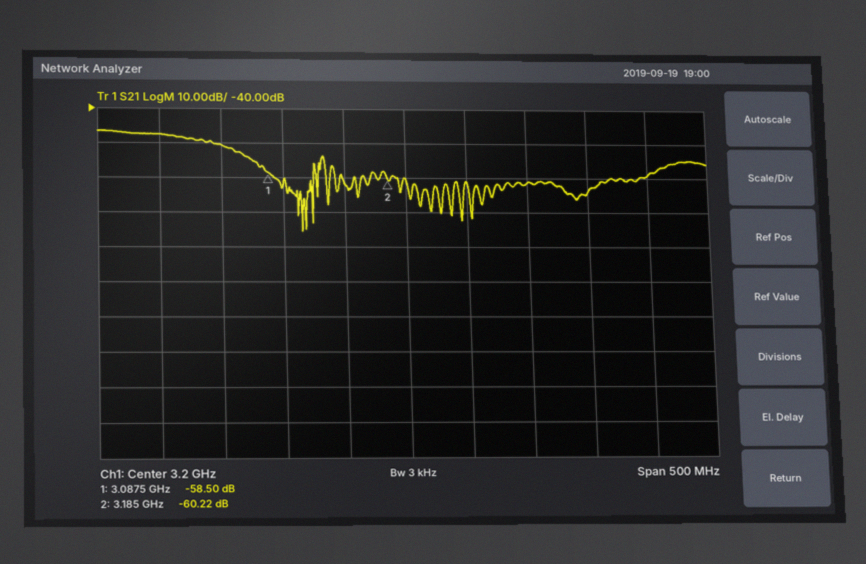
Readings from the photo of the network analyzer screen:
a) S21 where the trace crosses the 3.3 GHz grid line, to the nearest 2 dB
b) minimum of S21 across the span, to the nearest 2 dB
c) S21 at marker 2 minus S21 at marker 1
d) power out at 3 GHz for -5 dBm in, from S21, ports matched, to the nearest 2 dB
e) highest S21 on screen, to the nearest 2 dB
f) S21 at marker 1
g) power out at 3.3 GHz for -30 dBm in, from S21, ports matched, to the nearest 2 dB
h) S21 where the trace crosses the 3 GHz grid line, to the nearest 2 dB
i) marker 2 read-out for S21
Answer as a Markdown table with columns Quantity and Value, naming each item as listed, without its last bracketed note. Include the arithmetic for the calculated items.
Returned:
| Quantity | Value |
|---|---|
| S21 where the trace crosses the 3.3 GHz grid line, to the nearest 2 dB | -62 dB |
| minimum of S21 across the span, to the nearest 2 dB | -76 dB |
| S21 at marker 2 minus S21 at marker 1 | -60.22 − (-58.5) = -1.72 dB |
| power out at 3 GHz for -5 dBm in, from S21, ports matched, to the nearest 2 dB | -5 dBm + (-48 dB) = -52 dBm |
| highest S21 on screen, to the nearest 2 dB | -46 dB |
| S21 at marker 1 | -58.50 dB |
| power out at 3.3 GHz for -30 dBm in, from S21, ports matched, to the nearest 2 dB | -30 dBm + (-62 dB) = -92 dBm |
| S21 where the trace crosses the 3 GHz grid line, to the nearest 2 dB | -48 dB |
| marker 2 read-out for S21 | -60.22 dB |
